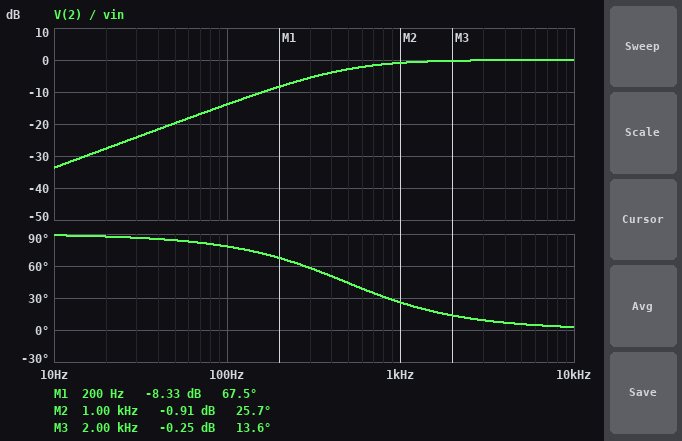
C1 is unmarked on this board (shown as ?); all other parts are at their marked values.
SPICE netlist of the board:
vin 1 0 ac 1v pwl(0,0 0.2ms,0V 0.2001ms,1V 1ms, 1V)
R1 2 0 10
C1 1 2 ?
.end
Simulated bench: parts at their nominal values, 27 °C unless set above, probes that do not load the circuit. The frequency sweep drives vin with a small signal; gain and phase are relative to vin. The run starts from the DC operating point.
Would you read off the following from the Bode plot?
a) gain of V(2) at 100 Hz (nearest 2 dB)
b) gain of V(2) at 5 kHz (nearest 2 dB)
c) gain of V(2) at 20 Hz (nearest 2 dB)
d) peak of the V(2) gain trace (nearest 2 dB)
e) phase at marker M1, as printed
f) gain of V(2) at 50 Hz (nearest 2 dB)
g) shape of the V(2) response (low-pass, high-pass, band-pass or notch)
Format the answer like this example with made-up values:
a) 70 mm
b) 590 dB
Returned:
a) -14 dB
b) 0 dB
c) -28 dB
d) 0 dB
e) 67.5 deg
f) -20 dB
g) high-pass
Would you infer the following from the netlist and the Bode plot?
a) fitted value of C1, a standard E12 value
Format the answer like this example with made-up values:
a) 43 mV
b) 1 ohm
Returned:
a) 33 µF
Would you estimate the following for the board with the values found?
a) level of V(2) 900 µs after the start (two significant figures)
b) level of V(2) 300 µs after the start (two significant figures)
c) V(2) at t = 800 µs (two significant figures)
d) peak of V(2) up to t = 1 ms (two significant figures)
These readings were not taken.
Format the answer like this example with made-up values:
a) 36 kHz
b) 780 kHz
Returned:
a) 120 mV
b) 740 mV
c) 160 mV
d) 1.0 V
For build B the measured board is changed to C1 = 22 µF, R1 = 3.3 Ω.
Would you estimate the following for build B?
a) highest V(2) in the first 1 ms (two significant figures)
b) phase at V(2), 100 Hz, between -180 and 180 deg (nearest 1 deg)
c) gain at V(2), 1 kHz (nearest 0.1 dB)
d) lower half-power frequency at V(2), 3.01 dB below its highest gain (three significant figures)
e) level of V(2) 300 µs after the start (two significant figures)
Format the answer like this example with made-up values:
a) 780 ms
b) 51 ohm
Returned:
a) 1.0 V
b) 87 deg
c) -7.6 dB
d) 2.19 kHz
e) 250 mV
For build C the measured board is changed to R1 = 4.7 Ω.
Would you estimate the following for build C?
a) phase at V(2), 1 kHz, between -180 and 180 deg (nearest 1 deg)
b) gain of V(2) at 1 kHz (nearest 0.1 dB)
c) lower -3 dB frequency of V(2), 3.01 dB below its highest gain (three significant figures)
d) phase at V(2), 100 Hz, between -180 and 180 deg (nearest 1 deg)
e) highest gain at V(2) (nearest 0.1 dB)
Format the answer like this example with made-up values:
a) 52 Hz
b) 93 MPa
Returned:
a) 46 deg
b) -3.1 dB
c) 1.03 kHz
d) 84 deg
e) 0 dB
